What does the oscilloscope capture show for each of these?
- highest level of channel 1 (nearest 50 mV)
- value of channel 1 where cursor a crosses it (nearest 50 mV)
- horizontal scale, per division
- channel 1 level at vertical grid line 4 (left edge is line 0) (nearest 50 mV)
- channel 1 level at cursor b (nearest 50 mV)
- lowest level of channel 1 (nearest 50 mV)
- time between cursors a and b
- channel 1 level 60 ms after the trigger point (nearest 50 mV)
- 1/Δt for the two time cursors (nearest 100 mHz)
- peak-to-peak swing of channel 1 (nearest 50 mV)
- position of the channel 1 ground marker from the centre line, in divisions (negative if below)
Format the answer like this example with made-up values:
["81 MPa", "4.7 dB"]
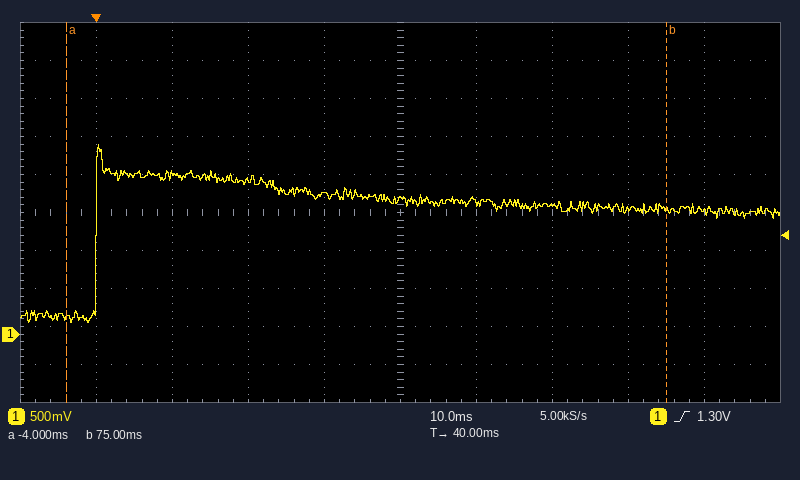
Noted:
["2.50 V", "200 mV", "10 ms", "1.85 V", "1.65 V", "150 mV", "79 ms", "1.70 V", "12.7 Hz", "2.35 V", "-3.2 div"]
